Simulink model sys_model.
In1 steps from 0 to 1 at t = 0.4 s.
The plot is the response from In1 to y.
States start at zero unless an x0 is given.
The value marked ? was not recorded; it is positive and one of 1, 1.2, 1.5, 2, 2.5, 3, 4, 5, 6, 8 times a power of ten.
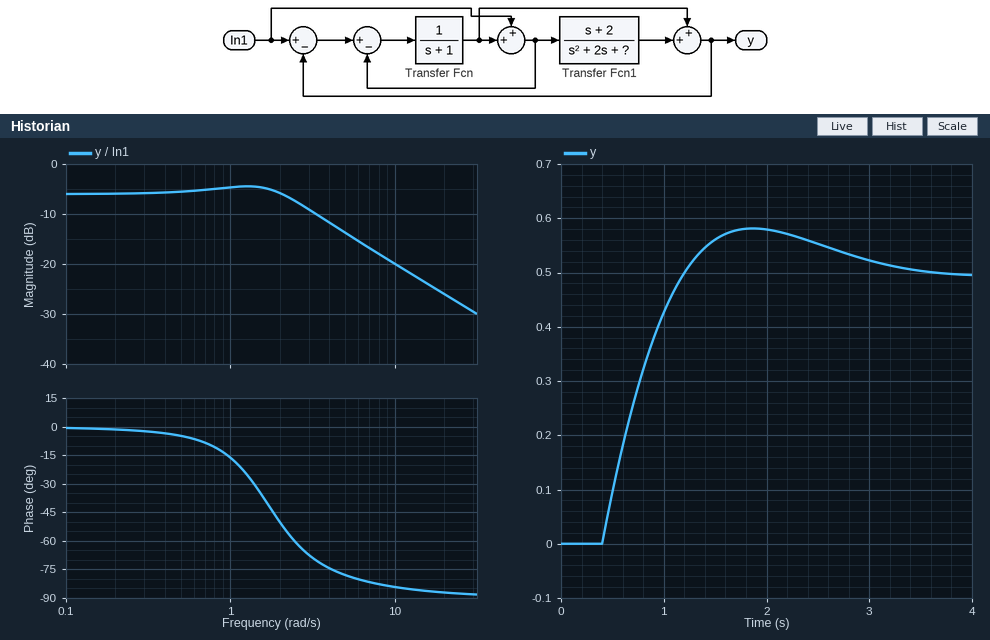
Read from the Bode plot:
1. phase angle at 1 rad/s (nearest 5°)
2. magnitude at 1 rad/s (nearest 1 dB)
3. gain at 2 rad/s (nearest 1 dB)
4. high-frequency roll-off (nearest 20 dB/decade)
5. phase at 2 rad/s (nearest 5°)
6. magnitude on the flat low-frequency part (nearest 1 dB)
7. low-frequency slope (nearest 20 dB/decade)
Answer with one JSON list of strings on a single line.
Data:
["-15°", "-5 dB", "-6 dB", "-20 dB/decade", "-50°", "-6 dB", "0 dB/decade"]
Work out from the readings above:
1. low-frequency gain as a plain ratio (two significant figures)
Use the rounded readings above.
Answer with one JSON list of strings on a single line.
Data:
["0.50"]
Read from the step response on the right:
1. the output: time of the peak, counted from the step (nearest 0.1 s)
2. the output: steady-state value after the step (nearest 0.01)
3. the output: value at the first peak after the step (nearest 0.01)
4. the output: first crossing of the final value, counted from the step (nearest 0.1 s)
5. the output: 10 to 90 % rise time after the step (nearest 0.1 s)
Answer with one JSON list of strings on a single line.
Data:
["1.5 s", "0.50", "0.58", "0.8 s", "0.6 s"]
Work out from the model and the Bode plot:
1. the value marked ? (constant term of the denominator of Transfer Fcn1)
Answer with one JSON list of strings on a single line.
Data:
["2"]
